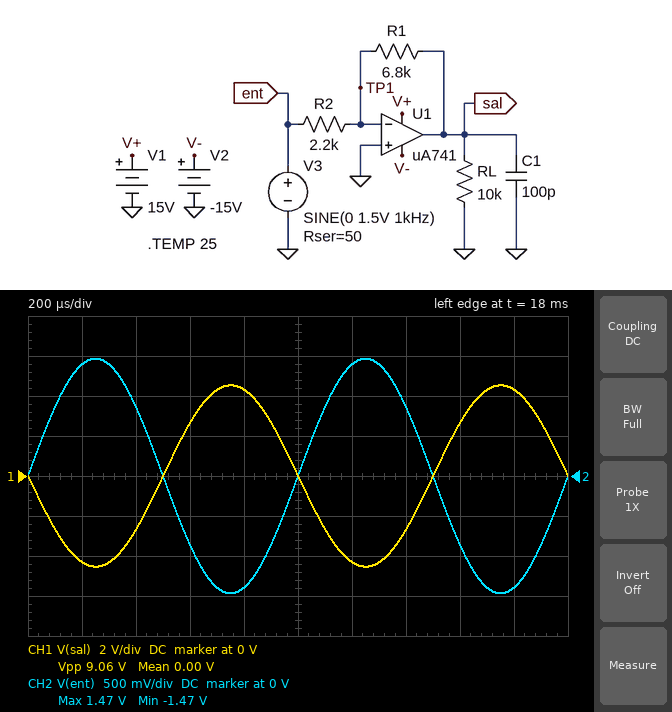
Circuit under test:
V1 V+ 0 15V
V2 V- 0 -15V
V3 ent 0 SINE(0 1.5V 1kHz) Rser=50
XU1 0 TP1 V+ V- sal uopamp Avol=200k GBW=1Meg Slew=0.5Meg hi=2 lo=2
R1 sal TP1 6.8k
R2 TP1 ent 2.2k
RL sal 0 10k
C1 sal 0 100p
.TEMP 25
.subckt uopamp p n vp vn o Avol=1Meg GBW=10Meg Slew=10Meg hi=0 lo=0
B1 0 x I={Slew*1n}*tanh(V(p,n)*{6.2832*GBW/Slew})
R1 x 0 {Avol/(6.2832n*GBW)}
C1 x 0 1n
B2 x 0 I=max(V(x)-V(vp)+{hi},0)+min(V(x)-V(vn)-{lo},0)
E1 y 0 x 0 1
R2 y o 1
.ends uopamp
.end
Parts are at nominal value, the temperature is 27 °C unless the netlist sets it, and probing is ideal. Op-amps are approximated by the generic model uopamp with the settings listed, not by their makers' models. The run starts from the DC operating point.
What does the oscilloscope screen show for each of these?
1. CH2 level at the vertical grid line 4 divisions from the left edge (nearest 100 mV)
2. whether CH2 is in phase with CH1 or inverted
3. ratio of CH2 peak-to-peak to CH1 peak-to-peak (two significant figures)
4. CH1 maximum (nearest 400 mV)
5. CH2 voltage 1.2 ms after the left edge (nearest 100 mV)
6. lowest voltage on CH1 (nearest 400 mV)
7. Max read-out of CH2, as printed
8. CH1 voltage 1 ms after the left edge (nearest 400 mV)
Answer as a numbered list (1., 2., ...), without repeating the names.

1. -1.4 V
2. inverted
3. 0.32
4. 4.4 V
5. 1.4 V
6. -4.4 V
7. 1.47 V
8. 0 V
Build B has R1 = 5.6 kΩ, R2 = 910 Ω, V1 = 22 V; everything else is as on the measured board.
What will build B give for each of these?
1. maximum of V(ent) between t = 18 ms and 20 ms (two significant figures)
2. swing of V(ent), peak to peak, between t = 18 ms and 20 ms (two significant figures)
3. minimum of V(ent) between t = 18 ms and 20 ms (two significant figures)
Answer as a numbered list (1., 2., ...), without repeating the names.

1. 1.4 V
2. 2.8 V
3. -1.4 V
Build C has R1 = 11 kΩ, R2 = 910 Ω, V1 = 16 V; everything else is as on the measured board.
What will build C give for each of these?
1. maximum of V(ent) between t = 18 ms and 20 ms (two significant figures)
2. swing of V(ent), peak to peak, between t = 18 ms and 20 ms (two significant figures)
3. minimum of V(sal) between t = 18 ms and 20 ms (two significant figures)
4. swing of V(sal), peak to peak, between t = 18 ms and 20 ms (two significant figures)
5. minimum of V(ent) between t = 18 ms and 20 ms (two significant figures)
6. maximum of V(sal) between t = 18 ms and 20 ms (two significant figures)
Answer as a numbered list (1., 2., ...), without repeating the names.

1. 1.4 V
2. 2.9 V
3. -13 V
4. 27 V
5. -1.4 V
6. 14 V
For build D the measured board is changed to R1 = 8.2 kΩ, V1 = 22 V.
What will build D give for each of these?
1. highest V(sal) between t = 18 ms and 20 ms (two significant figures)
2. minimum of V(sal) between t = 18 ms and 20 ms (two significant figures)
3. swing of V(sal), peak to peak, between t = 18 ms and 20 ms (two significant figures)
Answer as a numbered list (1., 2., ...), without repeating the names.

1. 5.5 V
2. -5.5 V
3. 11 V
